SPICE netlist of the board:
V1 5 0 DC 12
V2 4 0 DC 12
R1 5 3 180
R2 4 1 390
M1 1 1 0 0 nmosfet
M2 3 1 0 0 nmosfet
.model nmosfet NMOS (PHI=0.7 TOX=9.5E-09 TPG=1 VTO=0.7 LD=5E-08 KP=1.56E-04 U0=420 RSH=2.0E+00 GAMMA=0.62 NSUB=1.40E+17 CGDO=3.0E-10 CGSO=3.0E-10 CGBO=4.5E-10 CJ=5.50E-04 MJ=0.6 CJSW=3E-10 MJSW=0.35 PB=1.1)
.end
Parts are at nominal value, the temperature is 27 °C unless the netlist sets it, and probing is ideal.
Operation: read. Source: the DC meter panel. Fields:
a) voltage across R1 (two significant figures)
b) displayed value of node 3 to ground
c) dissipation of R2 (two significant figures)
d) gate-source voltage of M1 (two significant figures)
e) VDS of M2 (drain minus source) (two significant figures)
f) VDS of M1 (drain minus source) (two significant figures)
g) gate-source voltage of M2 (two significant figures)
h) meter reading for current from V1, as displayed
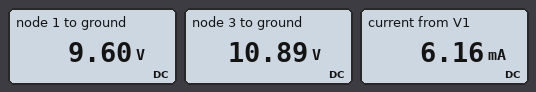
1.1 V
10.89 V
15 mW
9.6 V
11 V
9.6 V
9.6 V
6.16 mA
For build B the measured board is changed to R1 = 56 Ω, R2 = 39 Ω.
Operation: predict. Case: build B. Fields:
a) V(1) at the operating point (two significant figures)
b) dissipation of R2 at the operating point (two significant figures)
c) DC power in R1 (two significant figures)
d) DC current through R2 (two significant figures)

12 V
3.4 mW
4.8 mW
9.3 mA
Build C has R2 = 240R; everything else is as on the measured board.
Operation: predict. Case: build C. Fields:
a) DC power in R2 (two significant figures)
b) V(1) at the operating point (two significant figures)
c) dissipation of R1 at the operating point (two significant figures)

12 mW
10 V
9.2 mW
